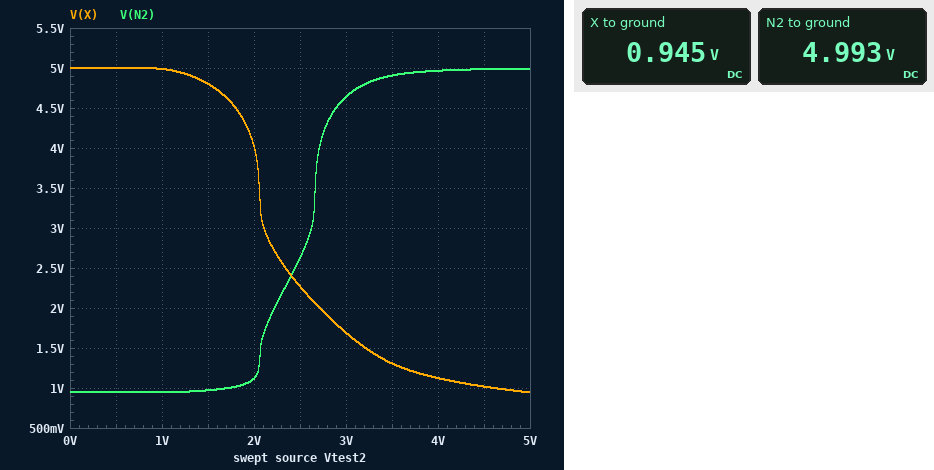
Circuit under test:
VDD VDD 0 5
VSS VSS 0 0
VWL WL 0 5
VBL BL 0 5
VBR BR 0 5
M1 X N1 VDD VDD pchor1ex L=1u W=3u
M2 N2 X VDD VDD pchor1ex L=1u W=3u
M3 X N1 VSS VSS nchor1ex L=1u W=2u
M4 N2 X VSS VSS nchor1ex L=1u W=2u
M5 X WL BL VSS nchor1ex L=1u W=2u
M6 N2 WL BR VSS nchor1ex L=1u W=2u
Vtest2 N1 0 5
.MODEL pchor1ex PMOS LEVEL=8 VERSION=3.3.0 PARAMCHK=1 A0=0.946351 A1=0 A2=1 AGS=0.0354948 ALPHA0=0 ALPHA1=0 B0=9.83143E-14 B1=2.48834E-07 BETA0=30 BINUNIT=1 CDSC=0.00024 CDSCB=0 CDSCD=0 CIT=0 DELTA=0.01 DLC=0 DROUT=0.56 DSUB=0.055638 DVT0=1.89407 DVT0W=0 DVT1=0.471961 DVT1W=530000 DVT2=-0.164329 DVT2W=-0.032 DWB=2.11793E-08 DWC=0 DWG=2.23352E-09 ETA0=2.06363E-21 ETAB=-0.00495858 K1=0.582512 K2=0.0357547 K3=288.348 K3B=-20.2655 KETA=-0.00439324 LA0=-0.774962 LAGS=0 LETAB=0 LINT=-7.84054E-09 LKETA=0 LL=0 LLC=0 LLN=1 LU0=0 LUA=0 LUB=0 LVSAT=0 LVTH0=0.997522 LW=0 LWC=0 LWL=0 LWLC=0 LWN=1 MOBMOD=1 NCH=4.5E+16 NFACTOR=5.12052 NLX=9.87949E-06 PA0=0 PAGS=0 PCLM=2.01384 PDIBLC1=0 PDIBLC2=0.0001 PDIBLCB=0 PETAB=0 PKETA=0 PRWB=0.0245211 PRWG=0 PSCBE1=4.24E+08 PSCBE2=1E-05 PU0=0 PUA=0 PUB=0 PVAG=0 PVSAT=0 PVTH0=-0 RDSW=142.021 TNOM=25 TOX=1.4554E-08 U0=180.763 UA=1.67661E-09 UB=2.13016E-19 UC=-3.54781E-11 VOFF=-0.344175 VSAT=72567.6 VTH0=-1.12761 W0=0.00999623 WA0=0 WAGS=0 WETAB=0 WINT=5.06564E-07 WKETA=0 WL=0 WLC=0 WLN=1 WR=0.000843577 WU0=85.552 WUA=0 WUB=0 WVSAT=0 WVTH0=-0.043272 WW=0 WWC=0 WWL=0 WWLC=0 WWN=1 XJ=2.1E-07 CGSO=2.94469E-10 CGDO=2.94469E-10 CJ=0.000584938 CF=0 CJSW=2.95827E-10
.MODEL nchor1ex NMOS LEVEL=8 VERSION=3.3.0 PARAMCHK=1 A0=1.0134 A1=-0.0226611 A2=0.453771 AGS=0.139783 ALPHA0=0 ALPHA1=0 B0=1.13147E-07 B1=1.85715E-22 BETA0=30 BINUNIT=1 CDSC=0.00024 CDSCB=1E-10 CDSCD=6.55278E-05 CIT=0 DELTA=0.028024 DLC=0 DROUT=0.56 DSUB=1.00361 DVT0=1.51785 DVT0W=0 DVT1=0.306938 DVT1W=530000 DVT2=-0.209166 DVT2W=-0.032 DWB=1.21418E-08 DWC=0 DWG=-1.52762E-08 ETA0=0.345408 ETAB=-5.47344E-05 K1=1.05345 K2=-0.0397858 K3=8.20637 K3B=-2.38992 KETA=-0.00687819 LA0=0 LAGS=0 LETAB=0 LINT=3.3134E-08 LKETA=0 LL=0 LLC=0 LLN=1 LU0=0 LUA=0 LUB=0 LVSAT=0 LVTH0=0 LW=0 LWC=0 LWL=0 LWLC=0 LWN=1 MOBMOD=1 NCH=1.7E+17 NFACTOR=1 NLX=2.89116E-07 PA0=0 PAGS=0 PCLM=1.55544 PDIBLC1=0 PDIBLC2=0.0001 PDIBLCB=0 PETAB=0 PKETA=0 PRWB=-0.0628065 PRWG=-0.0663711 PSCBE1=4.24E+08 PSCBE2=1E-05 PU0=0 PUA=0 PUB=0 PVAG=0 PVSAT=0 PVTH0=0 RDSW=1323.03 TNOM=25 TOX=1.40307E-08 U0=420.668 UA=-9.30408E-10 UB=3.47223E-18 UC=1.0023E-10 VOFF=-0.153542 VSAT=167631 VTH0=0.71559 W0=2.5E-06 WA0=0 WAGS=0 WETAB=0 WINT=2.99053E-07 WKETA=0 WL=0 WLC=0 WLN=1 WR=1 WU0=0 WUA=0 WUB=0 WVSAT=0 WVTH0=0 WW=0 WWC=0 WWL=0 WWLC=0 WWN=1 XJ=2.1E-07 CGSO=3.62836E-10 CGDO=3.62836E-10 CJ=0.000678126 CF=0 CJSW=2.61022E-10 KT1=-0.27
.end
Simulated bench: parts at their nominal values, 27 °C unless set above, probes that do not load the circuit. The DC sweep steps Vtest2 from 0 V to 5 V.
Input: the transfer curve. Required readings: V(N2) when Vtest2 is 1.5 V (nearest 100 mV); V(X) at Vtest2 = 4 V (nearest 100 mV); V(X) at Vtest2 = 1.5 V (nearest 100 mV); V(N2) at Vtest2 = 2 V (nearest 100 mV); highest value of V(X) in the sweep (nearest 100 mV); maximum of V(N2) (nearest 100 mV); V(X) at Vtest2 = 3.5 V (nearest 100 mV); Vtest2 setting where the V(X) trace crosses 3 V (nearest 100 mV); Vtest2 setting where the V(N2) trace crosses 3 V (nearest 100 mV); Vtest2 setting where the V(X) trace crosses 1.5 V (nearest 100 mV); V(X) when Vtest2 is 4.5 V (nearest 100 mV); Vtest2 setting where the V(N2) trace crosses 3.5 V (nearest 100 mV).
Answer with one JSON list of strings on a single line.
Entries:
["1.0 V", "1.1 V", "4.8 V", "1.1 V", "5.0 V", "5.0 V", "1.3 V", "2.1 V", "2.6 V", "3.2 V", "1.0 V", "2.7 V"]
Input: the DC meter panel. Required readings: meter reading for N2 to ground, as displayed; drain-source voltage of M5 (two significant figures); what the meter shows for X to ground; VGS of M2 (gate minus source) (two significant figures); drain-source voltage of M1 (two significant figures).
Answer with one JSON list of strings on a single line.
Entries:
["4.993 V", "-4.1 V", "0.945 V", "-4.1 V", "-4.1 V"]
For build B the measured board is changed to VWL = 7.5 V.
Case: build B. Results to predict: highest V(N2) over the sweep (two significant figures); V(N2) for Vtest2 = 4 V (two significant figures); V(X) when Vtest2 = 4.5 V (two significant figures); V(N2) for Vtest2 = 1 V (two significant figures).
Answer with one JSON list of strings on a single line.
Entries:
["4.6 V", "3.9 V", "2.4 V", "2.1 V"]
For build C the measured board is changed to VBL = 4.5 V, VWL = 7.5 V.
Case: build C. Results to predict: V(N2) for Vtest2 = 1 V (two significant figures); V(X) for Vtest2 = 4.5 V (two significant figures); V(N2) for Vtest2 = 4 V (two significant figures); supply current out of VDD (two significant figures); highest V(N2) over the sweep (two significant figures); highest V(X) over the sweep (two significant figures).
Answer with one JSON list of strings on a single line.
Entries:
["2.2 V", "2.3 V", "4.0 V", "37 µA", "4.6 V", "4.8 V"]
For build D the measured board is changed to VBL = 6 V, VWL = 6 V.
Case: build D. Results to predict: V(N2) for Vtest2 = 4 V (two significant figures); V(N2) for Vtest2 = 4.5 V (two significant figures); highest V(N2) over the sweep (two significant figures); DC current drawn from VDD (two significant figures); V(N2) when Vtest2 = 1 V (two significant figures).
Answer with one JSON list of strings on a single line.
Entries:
["4.7 V", "4.8 V", "4.9 V", "14 µA", "1.3 V"]
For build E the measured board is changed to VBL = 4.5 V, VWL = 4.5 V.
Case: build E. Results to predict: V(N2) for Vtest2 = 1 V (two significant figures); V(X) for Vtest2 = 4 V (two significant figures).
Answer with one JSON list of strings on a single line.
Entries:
["780 mV", "910 mV"]
